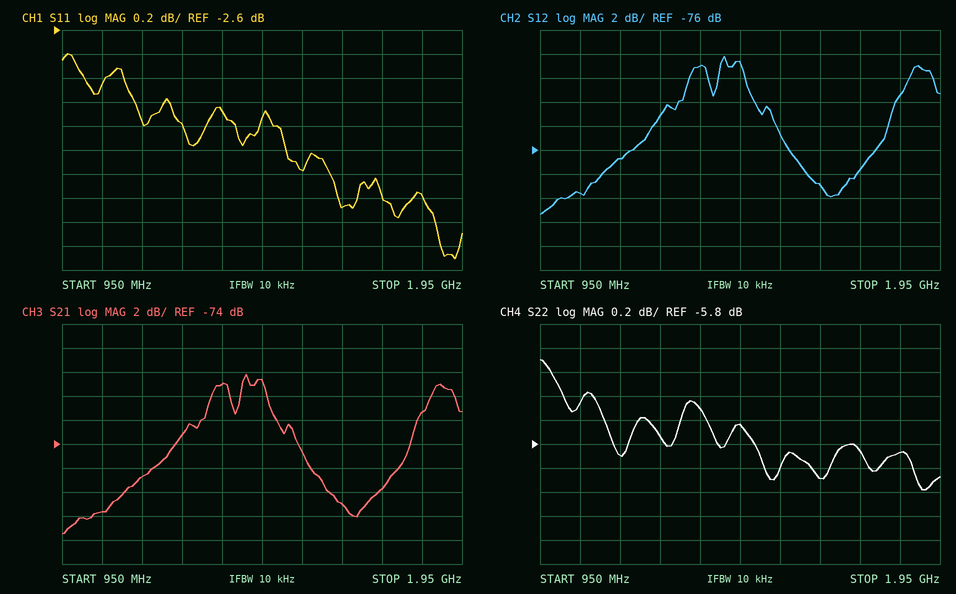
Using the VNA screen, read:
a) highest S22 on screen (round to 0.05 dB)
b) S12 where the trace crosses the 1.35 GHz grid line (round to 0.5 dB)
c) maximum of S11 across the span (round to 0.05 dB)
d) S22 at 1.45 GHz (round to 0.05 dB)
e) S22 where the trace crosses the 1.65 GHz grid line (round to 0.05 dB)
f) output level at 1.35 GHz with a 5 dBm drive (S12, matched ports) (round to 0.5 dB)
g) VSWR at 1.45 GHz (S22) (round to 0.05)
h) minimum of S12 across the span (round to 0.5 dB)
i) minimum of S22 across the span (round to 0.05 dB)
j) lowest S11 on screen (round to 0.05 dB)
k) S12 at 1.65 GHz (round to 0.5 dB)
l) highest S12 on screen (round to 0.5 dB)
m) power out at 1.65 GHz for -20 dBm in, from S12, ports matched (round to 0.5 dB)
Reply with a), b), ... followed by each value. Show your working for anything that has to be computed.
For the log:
a) -5.10 dB
b) -69.0 dB
c) -2.80 dB
d) -5.65 dB
e) -6.10 dB
f) 5 dBm + (-69.0 dB) = -64.0 dBm
g) |Γ| = 10^(-5.65/20) = 0.5218; VSWR = (1 + 0.5218)/(1 − 0.5218) ≈ 3.18, so 3.20 to the nearest 0.05
h) -81.5 dB
i) -6.20 dB
j) -4.50 dB
k) -79.0 dB
l) -68.0 dB
m) -20 dBm + (-79.0 dB) = -99.0 dBm
